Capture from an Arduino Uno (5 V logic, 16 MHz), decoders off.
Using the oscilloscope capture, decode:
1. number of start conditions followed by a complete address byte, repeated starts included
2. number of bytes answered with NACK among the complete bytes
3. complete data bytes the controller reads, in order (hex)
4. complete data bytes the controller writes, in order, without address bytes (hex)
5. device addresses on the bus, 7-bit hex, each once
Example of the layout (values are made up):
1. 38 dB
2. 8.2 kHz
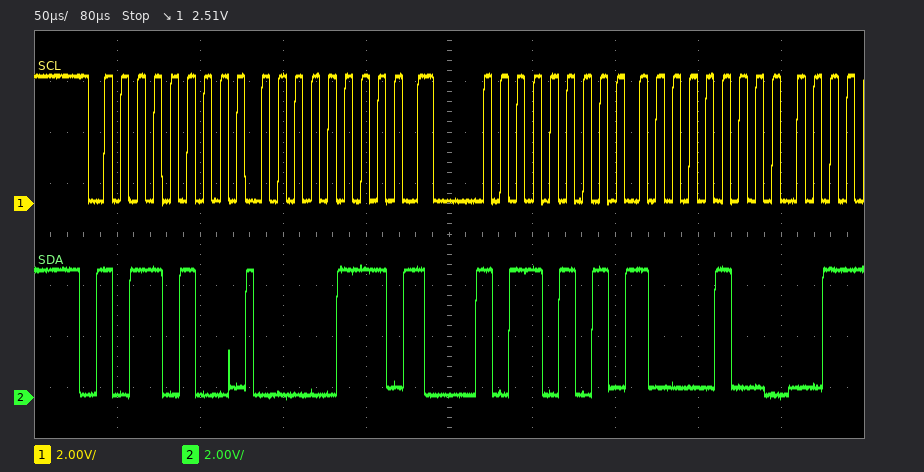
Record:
1. 2
2. 0
3. 84
4. 07
5. 0x5A
